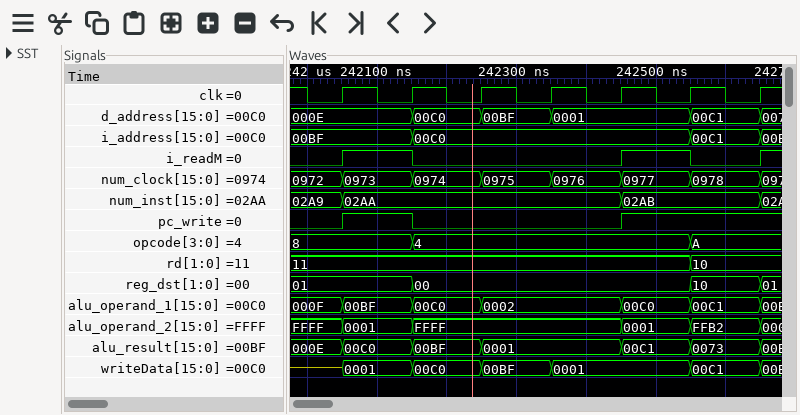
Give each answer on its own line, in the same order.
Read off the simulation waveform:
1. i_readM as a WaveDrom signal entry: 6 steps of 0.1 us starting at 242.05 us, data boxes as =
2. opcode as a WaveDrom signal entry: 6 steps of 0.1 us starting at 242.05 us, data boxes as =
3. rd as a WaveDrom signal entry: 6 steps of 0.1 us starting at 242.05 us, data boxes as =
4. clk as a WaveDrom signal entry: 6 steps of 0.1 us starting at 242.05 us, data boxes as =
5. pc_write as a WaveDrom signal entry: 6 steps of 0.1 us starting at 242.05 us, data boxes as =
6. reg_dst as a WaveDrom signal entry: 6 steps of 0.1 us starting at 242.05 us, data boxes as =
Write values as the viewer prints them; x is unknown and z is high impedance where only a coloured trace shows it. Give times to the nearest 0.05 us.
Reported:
{name: 'i_readM', wave: '10..10'}
{name: 'opcode', wave: '==...=', data: '8 4 A'}
{name: 'rd', wave: '=....=', data: '11 10'}
{name: 'clk', wave: 'p.....'}
{name: 'pc_write', wave: '10..1.'}
{name: 'reg_dst', wave: '==...=', data: '01 00 10'}
